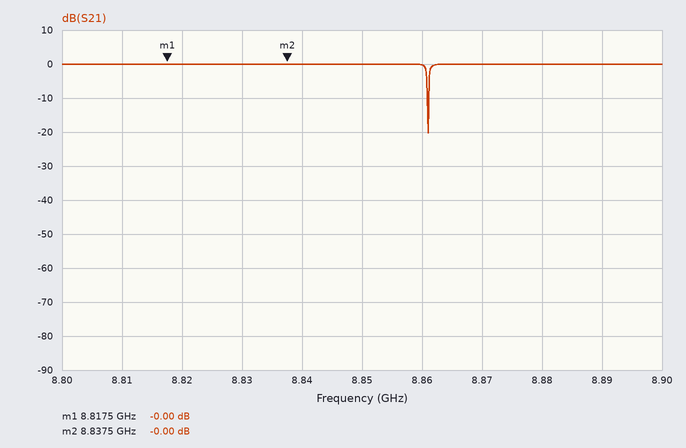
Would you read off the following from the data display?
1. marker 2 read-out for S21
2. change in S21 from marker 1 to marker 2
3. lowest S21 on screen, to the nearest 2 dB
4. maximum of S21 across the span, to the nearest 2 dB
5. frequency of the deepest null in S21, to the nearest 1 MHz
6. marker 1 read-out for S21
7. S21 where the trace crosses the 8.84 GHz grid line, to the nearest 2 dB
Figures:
-0.00 dB
0.00 dB
-20 dB
0 dB
8.861 GHz
-0.00 dB
0 dB
